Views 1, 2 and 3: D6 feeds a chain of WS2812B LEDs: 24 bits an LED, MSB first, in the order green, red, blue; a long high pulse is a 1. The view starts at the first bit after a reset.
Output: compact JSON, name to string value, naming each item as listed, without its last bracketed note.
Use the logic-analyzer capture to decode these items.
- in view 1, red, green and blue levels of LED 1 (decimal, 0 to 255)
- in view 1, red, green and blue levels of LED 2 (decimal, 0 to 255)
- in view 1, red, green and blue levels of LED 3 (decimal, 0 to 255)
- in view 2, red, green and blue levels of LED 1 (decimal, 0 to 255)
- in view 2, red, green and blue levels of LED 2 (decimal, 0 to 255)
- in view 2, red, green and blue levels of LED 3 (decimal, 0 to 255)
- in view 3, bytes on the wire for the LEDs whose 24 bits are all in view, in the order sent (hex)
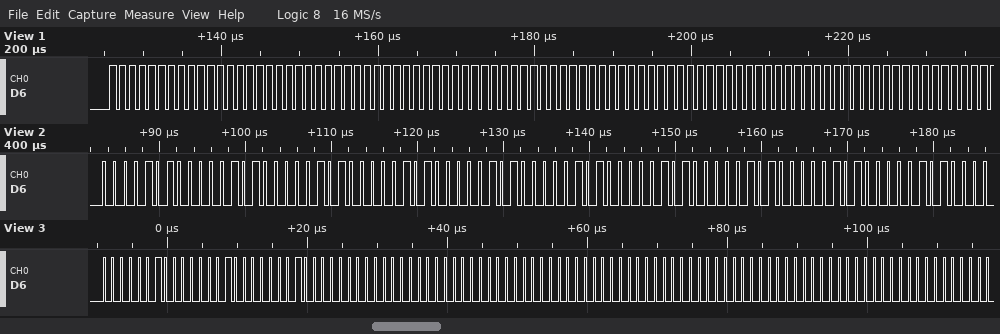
{"in view 1, red, green and blue levels of LED 1": "255, 255, 255", "in view 1, red, green and blue levels of LED 2": "255, 255, 255", "in view 1, red, green and blue levels of LED 3": "255, 255, 255", "in view 2, red, green and blue levels of LED 1": "10, 10, 10", "in view 2, red, green and blue levels of LED 2": "10, 10, 10", "in view 2, red, green and blue levels of LED 3": "10, 10, 10", "in view 3, bytes on the wire for the LEDs whose 24 bits are all in view, in the order sent": "02 02 02 00 00 00 00 00 00 00 00 00"}
